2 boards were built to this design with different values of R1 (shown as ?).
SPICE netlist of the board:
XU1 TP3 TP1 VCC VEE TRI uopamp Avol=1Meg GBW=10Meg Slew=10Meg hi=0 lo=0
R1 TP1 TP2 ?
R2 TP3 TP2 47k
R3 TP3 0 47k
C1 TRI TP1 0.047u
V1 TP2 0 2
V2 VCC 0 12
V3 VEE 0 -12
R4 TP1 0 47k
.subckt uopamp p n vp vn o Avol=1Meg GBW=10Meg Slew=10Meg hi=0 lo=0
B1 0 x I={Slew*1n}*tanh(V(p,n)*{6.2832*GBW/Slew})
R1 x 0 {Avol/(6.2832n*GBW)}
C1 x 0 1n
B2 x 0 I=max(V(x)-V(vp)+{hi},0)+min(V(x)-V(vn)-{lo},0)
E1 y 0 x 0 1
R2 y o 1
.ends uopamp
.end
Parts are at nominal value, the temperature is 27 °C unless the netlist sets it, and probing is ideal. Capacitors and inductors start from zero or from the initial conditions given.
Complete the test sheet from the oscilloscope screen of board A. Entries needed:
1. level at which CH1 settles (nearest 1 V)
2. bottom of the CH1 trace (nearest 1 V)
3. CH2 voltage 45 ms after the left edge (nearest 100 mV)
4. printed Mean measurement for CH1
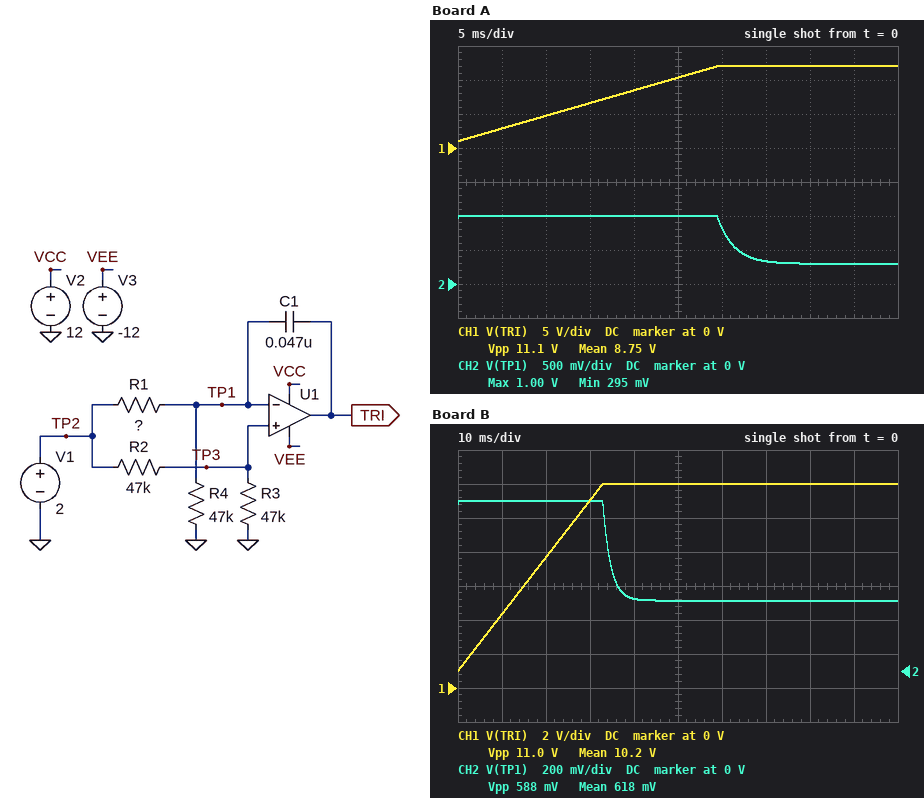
12 V
1 V
300 mV
8.75 V
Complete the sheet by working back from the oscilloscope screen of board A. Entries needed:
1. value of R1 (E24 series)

270 kΩ
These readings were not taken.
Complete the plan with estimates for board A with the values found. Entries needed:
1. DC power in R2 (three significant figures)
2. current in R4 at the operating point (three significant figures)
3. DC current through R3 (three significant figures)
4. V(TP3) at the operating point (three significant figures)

21.3 µW
6.31 µA
21.3 µA
1.00 V
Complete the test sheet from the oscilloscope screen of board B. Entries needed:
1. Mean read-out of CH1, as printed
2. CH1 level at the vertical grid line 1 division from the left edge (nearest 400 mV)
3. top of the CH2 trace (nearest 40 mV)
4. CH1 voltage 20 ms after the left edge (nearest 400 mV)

10.2 V
4.4 V
1.00 V
7.6 V
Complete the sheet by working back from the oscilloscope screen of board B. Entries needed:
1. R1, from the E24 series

180 kΩ
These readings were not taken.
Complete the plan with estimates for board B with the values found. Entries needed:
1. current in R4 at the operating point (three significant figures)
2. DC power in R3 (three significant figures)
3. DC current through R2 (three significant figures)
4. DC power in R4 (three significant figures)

8.81 µA
21.3 µW
21.3 µA
3.65 µW
